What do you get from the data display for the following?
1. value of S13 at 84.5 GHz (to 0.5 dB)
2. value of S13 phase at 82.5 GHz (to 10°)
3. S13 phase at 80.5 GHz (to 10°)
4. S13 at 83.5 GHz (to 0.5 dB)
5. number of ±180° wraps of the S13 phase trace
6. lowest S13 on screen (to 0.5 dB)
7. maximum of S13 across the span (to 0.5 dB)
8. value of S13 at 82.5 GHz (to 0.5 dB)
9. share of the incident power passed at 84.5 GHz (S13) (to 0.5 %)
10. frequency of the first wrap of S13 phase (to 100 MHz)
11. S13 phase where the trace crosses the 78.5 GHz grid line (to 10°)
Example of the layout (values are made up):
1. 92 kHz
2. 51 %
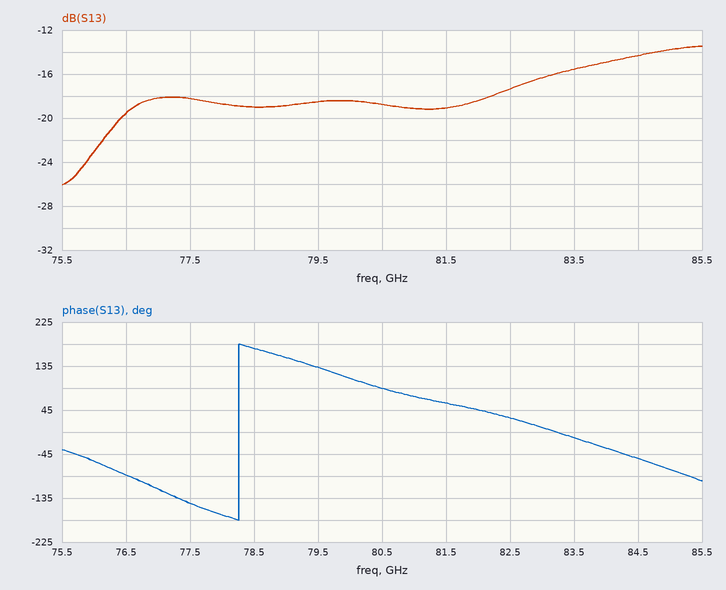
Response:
1. -14.5 dB
2. 30°
3. 90°
4. -15.5 dB
5. 1
6. -26.0 dB
7. -13.5 dB
8. -17.5 dB
9. 3.5 %
10. 78.3 GHz
11. 170°
